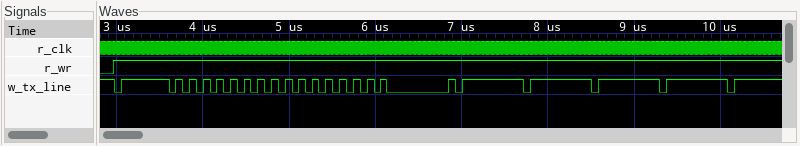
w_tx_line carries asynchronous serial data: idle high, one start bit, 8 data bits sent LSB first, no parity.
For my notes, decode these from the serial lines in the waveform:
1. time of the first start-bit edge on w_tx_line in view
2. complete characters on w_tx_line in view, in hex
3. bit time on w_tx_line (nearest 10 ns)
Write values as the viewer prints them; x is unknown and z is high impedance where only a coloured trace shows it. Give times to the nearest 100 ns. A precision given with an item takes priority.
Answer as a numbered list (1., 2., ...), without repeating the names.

1. 3000 ns
2. 7F, 55, 55, 55, 00, FF, FF, FF, FF
3. 80 ns
